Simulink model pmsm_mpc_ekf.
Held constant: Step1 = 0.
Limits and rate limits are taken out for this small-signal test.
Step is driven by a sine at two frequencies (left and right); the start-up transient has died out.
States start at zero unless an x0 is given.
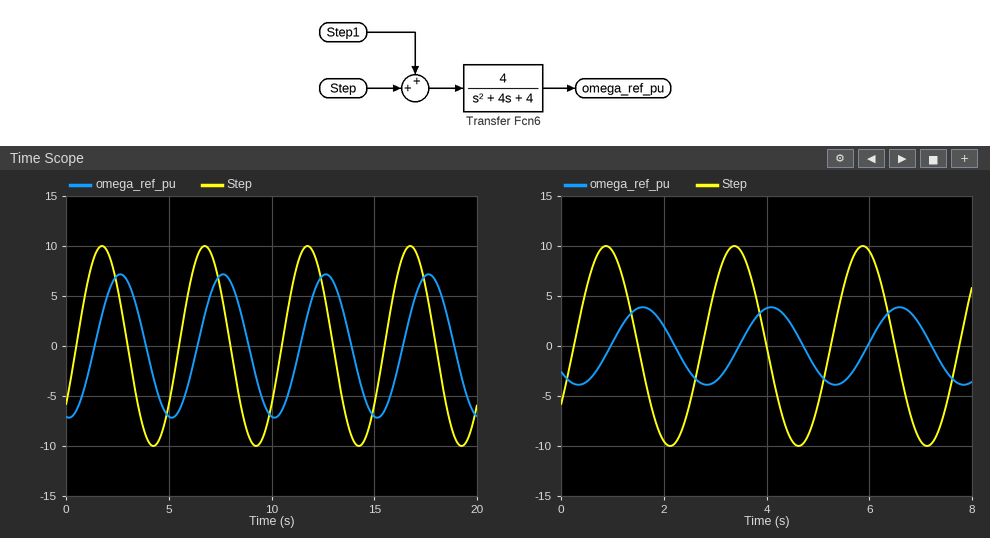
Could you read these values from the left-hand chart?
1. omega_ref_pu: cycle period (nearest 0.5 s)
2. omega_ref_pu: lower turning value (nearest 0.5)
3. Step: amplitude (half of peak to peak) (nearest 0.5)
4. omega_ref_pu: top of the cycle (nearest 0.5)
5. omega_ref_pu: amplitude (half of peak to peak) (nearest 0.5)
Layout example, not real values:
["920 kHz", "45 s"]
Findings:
["5.0 s", "-7.0", "10.0", "7.0", "7.0"]
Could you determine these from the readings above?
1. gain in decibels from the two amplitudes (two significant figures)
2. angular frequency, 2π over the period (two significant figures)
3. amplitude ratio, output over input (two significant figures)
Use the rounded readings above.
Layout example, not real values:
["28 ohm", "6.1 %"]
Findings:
["-3.1 dB", "1.3 rad/s", "0.70"]
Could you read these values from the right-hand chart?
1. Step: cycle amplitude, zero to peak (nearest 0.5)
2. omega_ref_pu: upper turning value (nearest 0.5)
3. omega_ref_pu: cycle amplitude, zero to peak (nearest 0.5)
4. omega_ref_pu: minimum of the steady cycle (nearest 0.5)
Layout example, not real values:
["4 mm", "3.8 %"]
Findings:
["10.0", "4.0", "4.0", "-4.0"]
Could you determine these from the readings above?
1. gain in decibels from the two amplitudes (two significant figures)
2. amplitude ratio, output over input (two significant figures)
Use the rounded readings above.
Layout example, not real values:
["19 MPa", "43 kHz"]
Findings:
["-8.0 dB", "0.40"]
